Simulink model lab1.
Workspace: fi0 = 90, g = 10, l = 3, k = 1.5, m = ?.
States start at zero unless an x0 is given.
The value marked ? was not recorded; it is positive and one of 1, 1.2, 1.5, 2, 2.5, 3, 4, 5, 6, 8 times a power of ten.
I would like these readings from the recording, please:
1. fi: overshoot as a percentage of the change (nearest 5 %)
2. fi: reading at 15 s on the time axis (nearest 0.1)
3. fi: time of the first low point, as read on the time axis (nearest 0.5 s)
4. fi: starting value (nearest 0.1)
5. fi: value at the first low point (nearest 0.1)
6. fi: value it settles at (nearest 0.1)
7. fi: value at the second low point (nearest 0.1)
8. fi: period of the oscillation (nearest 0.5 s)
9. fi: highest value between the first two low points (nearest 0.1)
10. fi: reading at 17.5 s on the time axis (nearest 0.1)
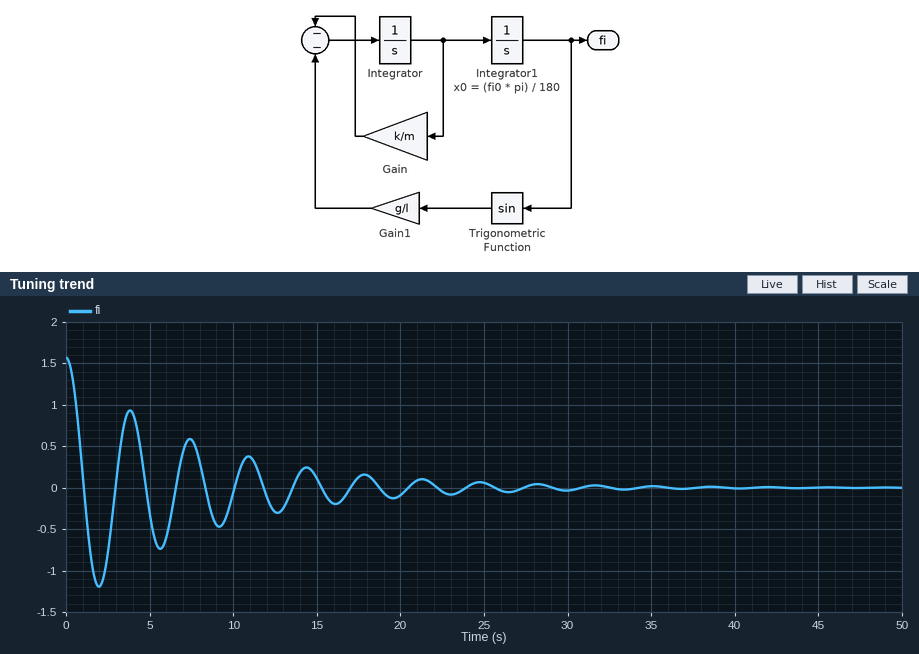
75 %
0.1
2.0 s
1.6
-1.2
0.0
-0.7
3.5 s
0.9
0.1
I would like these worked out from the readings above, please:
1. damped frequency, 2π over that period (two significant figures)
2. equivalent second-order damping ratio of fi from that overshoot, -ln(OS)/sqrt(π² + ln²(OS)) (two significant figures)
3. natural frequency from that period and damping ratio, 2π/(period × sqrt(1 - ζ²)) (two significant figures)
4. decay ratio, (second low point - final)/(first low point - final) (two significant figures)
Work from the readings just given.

1.8 rad/s
0.091
1.8 rad/s
0.58
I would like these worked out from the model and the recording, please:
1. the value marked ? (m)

6
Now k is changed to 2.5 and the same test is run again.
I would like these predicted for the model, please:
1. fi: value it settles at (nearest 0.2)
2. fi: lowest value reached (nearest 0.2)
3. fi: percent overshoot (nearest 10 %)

0.0
-1.0
60 %
